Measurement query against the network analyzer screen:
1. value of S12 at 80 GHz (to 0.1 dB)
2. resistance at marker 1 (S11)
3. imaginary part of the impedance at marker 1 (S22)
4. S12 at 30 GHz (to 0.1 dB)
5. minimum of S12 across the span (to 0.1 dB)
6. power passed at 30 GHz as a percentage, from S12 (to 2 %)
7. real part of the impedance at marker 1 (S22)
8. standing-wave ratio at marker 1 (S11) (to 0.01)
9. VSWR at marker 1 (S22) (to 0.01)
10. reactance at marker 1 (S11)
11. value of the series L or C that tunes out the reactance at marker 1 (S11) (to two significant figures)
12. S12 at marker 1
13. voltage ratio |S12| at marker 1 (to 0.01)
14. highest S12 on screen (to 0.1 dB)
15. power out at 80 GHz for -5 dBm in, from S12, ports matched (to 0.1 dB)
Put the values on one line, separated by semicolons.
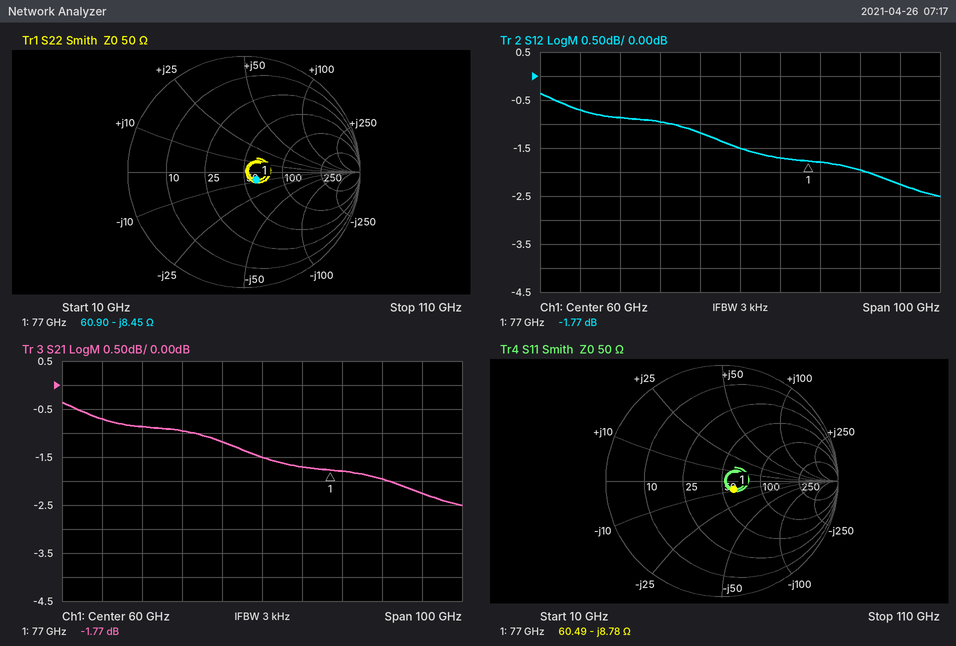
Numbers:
-1.8 dB; 60.49 Ω; -8.45 Ω; -0.9 dB; -2.5 dB; 82 %; 60.90 Ω; 1.28; 1.28; -8.78 Ω; 18 pH; -1.77 dB; 0.82; -0.4 dB; -6.8 dBm
